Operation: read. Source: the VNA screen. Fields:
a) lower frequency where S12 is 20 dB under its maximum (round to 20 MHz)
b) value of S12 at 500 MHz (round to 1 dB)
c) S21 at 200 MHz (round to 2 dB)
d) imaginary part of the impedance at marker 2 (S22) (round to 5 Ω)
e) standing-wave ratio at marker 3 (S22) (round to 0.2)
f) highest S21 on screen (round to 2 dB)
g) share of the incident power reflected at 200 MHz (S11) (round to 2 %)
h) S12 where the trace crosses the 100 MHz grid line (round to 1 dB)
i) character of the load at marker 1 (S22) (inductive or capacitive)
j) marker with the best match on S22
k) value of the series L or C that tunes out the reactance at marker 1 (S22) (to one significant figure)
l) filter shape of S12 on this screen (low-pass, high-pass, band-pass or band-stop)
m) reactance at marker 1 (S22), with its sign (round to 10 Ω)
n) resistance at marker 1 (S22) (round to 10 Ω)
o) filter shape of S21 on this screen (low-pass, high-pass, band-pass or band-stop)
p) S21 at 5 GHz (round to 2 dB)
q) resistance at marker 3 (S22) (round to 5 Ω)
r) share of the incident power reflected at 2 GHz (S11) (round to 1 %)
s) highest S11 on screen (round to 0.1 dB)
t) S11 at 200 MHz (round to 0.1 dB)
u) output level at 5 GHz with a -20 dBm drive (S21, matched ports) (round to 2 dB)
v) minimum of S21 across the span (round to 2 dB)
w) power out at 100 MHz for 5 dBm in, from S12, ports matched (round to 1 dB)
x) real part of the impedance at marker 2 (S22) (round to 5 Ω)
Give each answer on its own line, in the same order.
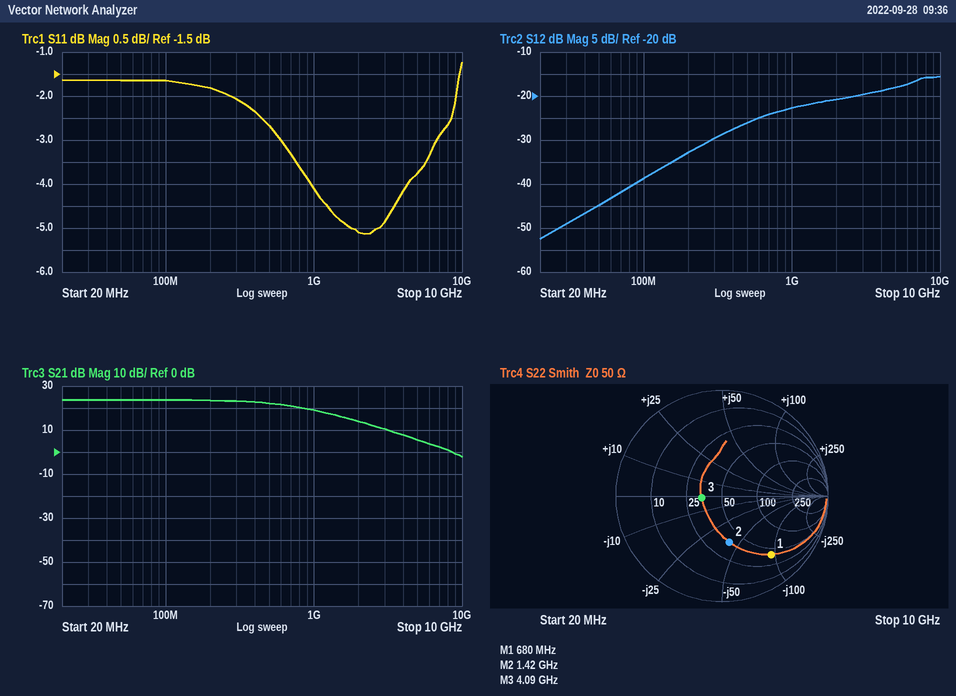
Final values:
140 MHz
-26 dB
24 dB
-40 Ω
1.4
24 dB
66 %
-39 dB
capacitive
marker 3
20 nH
high-pass
-90 Ω
40 Ω
low-pass
6 dB
35 Ω
31 %
-1.2 dB
-1.8 dB
-14 dBm
-2 dB
-34 dBm
40 Ω
